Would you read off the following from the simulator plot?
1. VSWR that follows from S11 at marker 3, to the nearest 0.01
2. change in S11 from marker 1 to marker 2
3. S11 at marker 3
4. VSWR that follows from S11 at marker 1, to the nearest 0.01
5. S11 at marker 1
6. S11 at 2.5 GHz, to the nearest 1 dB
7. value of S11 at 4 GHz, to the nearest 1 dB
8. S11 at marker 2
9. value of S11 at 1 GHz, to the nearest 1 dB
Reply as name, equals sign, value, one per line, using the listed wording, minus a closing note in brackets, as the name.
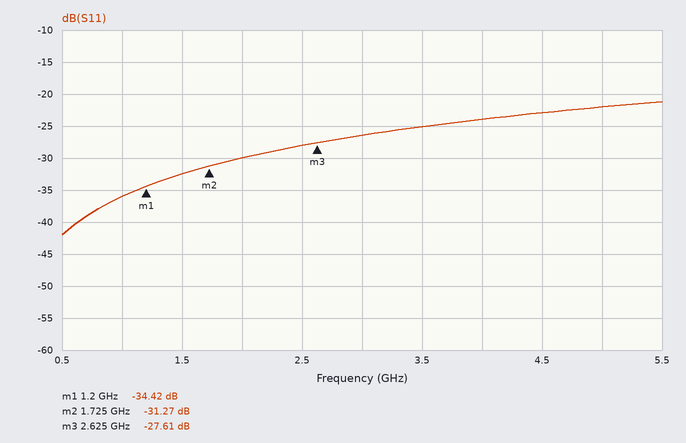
VSWR that follows from S11 at marker 3, to the nearest 0.01 = 1.09
change in S11 from marker 1 to marker 2 = 3.15 dB
S11 at marker 3 = -27.61 dB
VSWR that follows from S11 at marker 1, to the nearest 0.01 = 1.04
S11 at marker 1 = -34.42 dB
S11 at 2.5 GHz, to the nearest 1 dB = -28 dB
value of S11 at 4 GHz, to the nearest 1 dB = -24 dB
S11 at marker 2 = -31.27 dB
value of S11 at 1 GHz, to the nearest 1 dB = -36 dB
